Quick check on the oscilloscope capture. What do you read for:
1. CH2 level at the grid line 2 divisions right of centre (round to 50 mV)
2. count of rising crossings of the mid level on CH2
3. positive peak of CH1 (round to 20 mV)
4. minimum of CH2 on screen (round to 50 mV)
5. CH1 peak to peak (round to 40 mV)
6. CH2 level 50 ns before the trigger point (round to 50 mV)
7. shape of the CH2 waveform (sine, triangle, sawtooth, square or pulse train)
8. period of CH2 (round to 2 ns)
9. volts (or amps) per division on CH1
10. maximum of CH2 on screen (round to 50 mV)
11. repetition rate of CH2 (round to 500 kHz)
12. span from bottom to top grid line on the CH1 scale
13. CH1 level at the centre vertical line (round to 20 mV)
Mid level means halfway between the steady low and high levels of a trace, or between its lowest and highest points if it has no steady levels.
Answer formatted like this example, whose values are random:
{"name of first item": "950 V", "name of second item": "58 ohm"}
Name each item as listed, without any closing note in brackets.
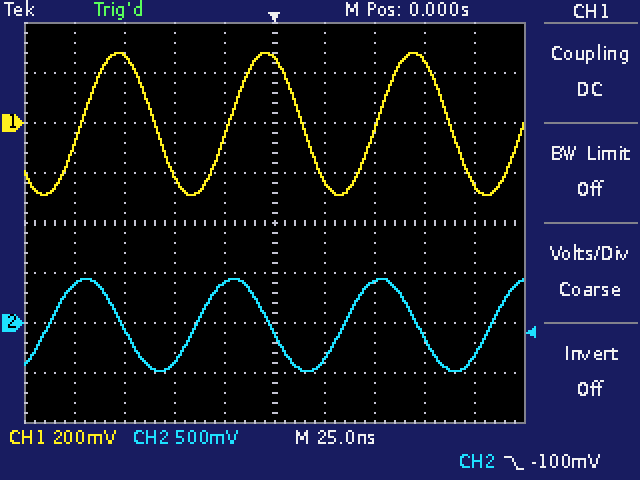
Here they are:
{"CH2 level at the grid line 2 divisions right of centre": "400 mV", "count of rising crossings of the mid level on CH2": "4", "positive peak of CH1": "280 mV", "minimum of CH2 on screen": "-500 mV", "CH1 peak to peak": "560 mV", "CH2 level 50 ns before the trigger point": "-400 mV", "shape of the CH2 waveform": "sine", "period of CH2": "74 ns", "volts (or amps) per division on CH1": "200 mV", "maximum of CH2 on screen": "450 mV", "repetition rate of CH2": "13.5 MHz", "span from bottom to top grid line on the CH1 scale": "1.6 V", "CH1 level at the centre vertical line": "260 mV"}
